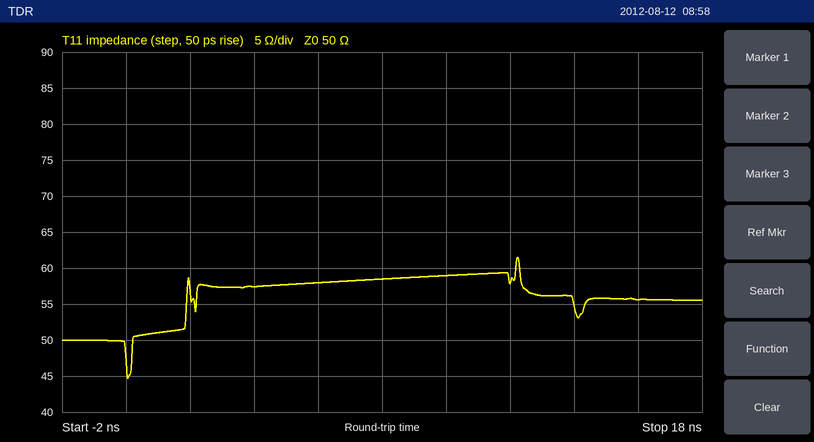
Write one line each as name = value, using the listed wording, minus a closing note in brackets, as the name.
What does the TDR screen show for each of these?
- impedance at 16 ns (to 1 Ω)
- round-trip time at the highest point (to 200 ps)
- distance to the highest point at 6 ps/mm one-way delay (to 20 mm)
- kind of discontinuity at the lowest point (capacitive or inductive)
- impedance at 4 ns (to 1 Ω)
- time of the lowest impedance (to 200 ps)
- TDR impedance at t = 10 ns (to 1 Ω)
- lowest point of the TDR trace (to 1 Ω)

impedance at 16 ns = 56 Ω
round-trip time at the highest point = 12.2 ns
distance to the highest point at 6 ps/mm one-way delay = 1.02 m
kind of discontinuity at the lowest point = capacitive
impedance at 4 ns = 57 Ω
time of the lowest impedance = 0.0 ns
TDR impedance at t = 10 ns = 59 Ω
lowest point of the TDR trace = 45 Ω
